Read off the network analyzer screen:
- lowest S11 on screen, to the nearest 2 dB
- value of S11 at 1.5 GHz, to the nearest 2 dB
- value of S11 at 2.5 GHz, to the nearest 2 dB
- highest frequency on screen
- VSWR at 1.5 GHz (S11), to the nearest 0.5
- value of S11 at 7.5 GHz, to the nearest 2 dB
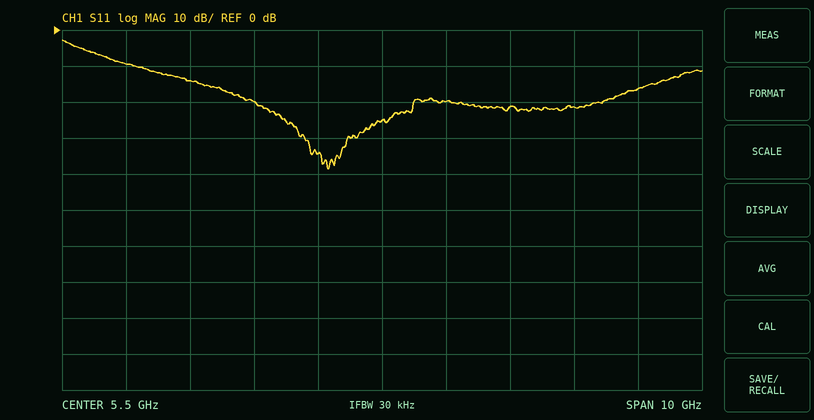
-38 dB
-10 dB
-14 dB
10.5 GHz
2.0
-22 dB
